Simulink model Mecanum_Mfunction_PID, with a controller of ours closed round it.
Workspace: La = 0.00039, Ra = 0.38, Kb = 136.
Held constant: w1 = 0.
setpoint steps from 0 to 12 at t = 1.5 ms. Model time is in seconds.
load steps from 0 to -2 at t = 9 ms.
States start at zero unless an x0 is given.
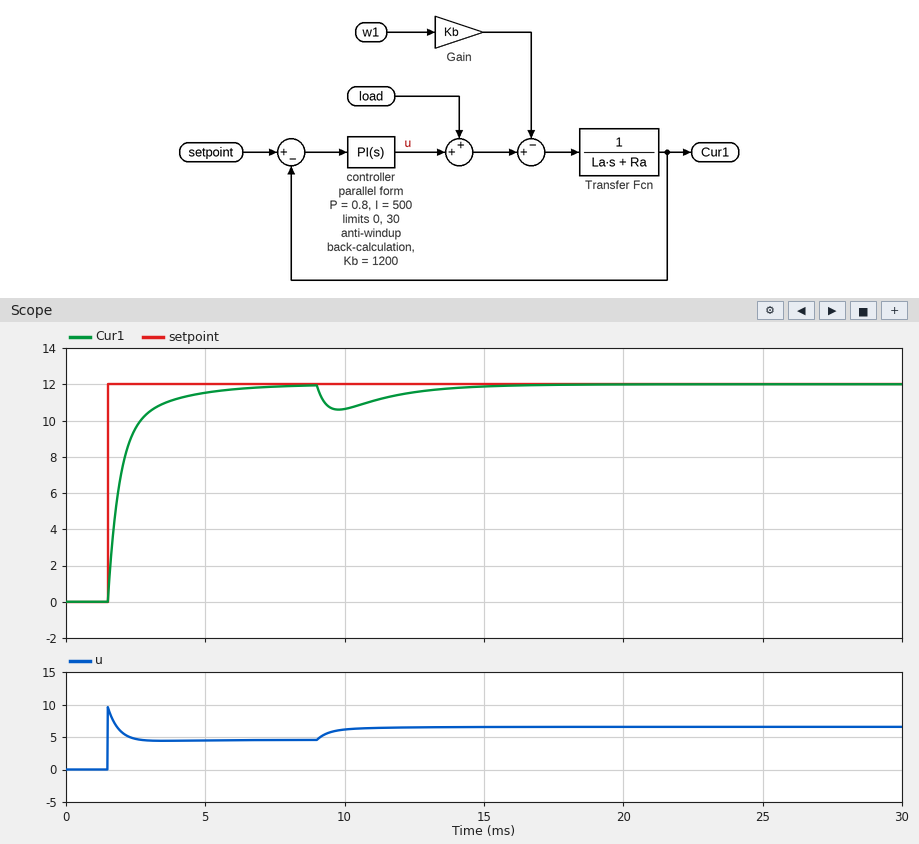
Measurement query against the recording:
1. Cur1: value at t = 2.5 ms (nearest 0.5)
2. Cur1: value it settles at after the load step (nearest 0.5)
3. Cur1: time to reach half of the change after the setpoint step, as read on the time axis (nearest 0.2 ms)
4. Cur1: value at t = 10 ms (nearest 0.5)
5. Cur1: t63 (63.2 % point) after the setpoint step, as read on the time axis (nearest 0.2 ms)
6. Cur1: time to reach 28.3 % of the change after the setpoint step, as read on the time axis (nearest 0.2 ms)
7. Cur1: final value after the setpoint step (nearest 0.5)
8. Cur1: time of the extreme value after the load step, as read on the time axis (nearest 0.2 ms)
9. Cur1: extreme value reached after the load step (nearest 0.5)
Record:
9.5
12.0
1.8 ms
10.5
2.0 ms
1.6 ms
12.0
9.8 ms
10.5
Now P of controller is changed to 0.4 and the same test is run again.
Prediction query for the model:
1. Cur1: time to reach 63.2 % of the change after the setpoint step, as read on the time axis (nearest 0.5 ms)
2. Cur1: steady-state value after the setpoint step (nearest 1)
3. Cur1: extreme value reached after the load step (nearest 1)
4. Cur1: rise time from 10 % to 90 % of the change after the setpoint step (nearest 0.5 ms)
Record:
2.5 ms
12
10
1.5 ms
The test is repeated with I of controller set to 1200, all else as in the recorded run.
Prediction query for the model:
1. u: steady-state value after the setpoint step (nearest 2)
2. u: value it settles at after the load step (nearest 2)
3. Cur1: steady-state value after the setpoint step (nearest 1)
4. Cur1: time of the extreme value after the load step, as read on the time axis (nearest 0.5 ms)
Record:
4
6
12
9.5 ms
